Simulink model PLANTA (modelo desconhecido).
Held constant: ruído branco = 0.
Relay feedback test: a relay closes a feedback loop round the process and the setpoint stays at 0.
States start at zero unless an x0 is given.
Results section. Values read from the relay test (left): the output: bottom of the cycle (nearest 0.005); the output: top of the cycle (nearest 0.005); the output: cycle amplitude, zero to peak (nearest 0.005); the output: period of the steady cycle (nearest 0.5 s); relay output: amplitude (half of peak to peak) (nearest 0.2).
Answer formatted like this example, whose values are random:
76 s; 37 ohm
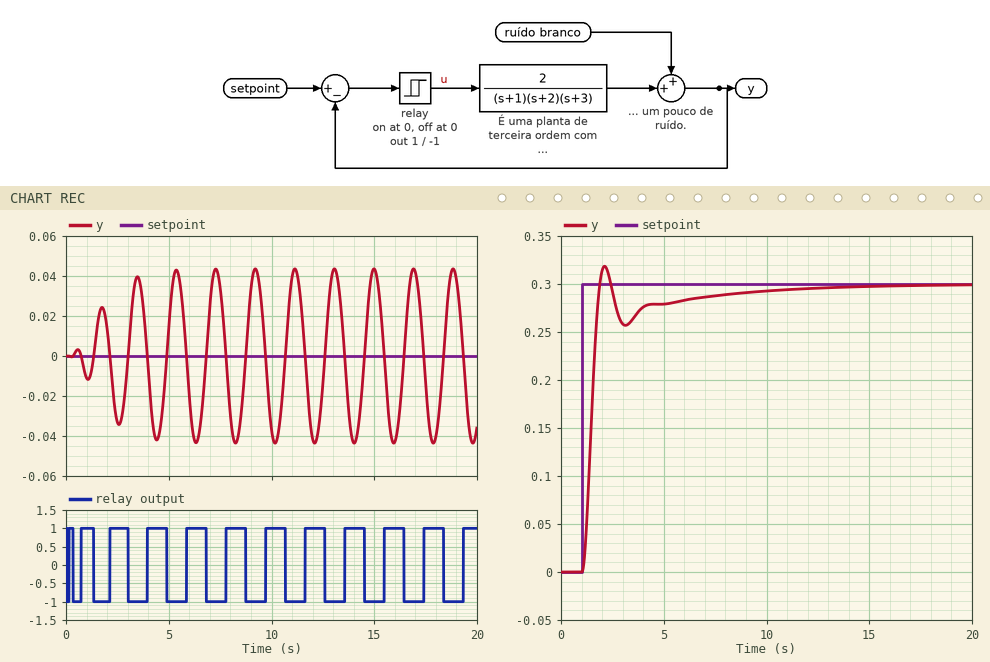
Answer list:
-0.045; 0.045; 0.045; 2.0 s; 1.0
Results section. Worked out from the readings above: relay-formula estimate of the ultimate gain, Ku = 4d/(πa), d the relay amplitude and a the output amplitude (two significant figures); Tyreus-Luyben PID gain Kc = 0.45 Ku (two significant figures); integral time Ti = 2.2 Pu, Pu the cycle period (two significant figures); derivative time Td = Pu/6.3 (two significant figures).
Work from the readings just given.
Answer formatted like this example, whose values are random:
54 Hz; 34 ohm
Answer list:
28; 13; 4.4 s; 0.32 s
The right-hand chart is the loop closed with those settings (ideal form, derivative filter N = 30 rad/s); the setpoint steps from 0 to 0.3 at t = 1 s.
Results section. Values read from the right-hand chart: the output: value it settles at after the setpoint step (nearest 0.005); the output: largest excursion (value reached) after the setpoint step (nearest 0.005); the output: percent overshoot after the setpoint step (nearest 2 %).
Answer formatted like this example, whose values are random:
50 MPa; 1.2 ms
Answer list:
0.300; 0.320; 6 %
